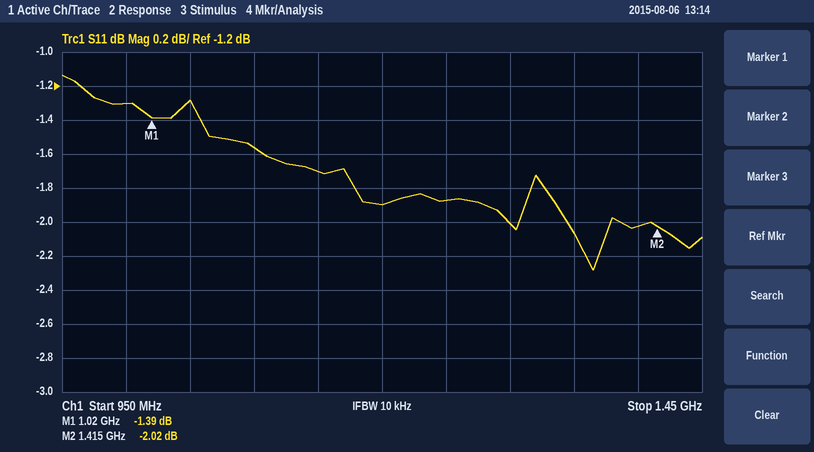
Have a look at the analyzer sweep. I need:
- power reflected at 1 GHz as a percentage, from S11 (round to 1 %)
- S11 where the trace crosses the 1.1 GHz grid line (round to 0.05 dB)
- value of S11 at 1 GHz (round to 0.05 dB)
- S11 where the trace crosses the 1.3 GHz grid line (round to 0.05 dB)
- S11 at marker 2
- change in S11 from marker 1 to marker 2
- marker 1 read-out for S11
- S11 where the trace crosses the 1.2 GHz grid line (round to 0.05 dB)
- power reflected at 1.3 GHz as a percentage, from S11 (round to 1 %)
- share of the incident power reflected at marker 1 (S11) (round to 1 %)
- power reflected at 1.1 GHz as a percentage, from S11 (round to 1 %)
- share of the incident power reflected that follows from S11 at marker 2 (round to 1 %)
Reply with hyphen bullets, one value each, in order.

- 74 %
- -1.55 dB
- -1.30 dB
- -2.00 dB
- -2.02 dB
- -0.63 dB
- -1.39 dB
- -1.90 dB
- 63 %
- 73 %
- 70 %
- 63 %
